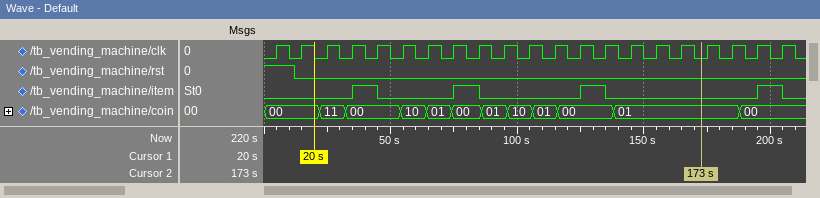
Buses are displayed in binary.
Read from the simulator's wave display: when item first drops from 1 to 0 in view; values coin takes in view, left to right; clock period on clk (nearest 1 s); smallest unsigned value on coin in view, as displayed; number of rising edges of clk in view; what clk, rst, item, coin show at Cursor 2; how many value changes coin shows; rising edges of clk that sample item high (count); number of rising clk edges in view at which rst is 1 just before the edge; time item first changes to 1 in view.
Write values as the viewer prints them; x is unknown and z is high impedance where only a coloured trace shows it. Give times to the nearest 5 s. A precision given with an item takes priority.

45 s
00, 11, 00, 10, 01, 00, 01, 10, 01, 00, 01, 00
10 s
00
21
clk=0, rst=0, item=0, coin=01
11
4
1
35 s
